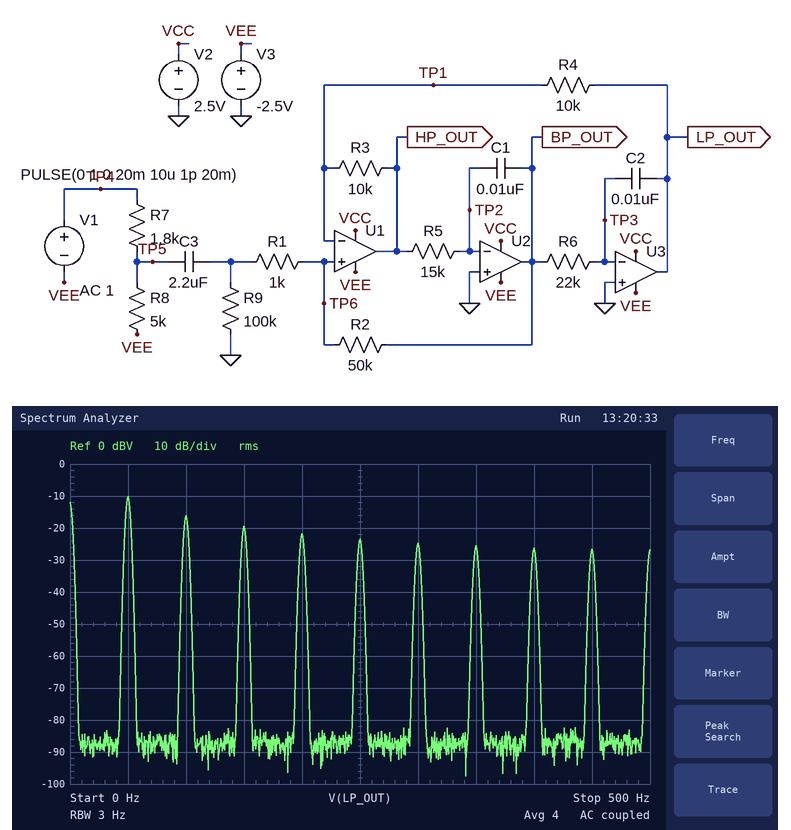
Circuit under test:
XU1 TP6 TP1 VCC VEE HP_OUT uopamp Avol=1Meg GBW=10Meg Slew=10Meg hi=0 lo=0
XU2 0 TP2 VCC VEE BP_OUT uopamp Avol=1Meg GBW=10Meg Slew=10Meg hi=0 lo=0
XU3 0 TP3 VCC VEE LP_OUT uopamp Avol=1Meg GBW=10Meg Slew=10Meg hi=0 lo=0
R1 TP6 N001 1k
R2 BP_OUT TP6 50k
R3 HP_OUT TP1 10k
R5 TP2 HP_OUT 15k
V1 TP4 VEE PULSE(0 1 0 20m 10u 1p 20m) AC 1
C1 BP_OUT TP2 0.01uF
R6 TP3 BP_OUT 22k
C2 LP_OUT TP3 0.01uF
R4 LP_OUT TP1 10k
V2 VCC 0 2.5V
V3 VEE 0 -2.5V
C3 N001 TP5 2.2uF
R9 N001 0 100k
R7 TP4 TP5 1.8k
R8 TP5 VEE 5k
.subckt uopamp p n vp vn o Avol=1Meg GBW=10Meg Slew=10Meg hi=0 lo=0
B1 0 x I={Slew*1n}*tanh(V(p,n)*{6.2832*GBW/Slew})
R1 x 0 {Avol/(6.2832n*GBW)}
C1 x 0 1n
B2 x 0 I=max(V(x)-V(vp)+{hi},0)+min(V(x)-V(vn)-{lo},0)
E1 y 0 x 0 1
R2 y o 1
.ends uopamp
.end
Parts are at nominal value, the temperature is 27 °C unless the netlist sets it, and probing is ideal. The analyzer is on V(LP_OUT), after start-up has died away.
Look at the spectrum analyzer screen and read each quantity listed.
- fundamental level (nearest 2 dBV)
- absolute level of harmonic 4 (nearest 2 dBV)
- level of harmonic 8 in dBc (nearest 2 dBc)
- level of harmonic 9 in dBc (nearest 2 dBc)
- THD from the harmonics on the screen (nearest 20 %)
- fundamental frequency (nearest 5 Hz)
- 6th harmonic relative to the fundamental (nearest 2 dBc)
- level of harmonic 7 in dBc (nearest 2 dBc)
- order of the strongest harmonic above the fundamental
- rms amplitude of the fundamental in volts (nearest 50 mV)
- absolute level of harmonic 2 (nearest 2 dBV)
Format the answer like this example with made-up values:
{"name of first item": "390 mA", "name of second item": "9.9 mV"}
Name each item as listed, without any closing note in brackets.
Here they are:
{"fundamental level": "-10 dBV", "absolute level of harmonic 4": "-22 dBV", "level of harmonic 8 in dBc": "-16 dBc", "level of harmonic 9 in dBc": "-16 dBc", "THD from the harmonics on the screen": "80 %", "fundamental frequency": "50 Hz", "6th harmonic relative to the fundamental": "-14 dBc", "level of harmonic 7 in dBc": "-16 dBc", "order of the strongest harmonic above the fundamental": "2", "rms amplitude of the fundamental in volts": "300 mV", "absolute level of harmonic 2": "-16 dBV"}
